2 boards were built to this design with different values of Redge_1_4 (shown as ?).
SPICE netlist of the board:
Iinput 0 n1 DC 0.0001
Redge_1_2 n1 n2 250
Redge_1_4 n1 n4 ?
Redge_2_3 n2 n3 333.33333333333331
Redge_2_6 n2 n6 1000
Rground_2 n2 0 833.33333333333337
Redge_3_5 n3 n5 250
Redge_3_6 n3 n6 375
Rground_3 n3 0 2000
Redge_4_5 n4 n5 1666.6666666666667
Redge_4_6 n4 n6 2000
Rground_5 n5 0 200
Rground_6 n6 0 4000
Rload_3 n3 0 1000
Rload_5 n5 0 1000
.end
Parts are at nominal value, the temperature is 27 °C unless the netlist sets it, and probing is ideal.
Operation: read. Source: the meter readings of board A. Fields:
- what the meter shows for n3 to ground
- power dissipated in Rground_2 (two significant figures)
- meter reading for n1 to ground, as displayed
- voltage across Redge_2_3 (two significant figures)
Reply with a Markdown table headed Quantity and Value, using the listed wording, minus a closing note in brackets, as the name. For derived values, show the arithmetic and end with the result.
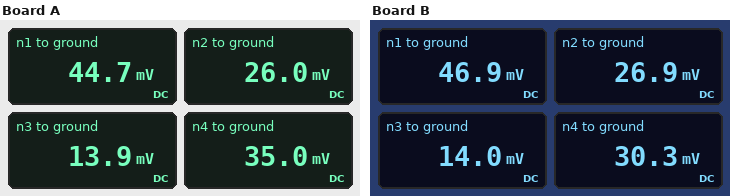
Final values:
| Quantity | Value |
|---|---|
| what the meter shows for n3 to ground | 13.9 mV |
| power dissipated in Rground_2 | (26 mV)^2 / 833.3 Ω = 810 nW |
| meter reading for n1 to ground, as displayed | 44.7 mV |
| voltage across Redge_2_3 | 26 mV - 13.9 mV = 12 mV |
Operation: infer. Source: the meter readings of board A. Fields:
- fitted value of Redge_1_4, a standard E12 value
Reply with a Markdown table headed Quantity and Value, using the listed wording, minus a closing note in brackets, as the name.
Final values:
| Quantity | Value |
|---|---|
| fitted value of Redge_1_4, a standard E12 value | 390 Ω |
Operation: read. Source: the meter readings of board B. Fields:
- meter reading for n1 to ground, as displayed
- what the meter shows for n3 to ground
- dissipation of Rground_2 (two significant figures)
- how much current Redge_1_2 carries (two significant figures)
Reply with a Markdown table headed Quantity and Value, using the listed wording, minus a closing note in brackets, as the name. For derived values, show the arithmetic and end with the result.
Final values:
| Quantity | Value |
|---|---|
| meter reading for n1 to ground, as displayed | 46.9 mV |
| what the meter shows for n3 to ground | 14.0 mV |
| dissipation of Rground_2 | (26.9 mV)^2 / 833.3 Ω = 870 nW |
| how much current Redge_1_2 carries | (46.9 mV - 26.9 mV) / 250 Ω = 80 µA |
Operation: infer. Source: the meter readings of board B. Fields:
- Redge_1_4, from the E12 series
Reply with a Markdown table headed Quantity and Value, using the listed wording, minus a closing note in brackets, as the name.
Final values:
| Quantity | Value |
|---|---|
| Redge_1_4, from the E12 series | 820 Ω |
